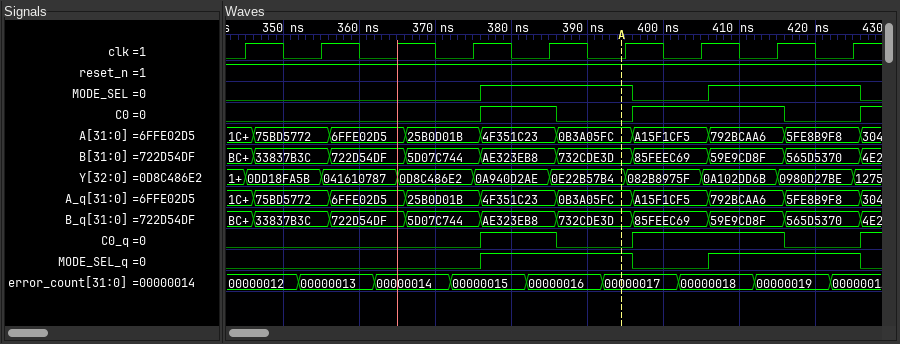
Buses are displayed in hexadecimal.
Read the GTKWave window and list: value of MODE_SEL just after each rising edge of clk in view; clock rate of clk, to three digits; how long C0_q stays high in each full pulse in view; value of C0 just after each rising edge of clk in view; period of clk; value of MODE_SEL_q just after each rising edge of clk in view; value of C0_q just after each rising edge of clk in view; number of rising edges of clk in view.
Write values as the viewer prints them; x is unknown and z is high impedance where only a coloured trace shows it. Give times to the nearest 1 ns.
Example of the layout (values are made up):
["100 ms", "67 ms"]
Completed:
["0 0 0 0 1 1 0 1 1", "100 MHz", "10 ns, 20 ns", "0 0 0 0 1 0 1 1 0", "10 ns", "0 0 0 0 1 1 0 1 1", "0 0 0 0 1 0 1 1 0", "9"]
